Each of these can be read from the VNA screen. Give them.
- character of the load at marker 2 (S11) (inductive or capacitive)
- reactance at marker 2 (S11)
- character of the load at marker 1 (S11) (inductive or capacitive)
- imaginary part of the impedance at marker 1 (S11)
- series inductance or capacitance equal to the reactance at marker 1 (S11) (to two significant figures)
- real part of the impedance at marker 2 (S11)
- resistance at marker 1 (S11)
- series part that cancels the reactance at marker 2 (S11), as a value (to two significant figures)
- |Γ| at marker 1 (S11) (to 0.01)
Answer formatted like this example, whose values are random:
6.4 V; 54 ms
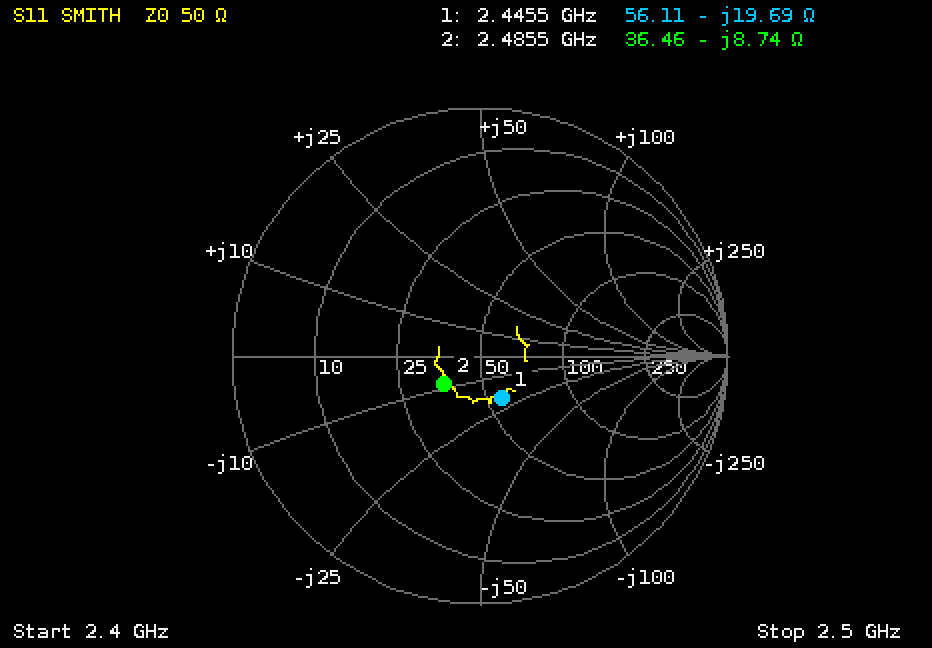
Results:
capacitive; -8.74 Ω; capacitive; -19.69 Ω; 3.3 pF; 36.46 Ω; 56.11 Ω; 560 pH; 0.19
